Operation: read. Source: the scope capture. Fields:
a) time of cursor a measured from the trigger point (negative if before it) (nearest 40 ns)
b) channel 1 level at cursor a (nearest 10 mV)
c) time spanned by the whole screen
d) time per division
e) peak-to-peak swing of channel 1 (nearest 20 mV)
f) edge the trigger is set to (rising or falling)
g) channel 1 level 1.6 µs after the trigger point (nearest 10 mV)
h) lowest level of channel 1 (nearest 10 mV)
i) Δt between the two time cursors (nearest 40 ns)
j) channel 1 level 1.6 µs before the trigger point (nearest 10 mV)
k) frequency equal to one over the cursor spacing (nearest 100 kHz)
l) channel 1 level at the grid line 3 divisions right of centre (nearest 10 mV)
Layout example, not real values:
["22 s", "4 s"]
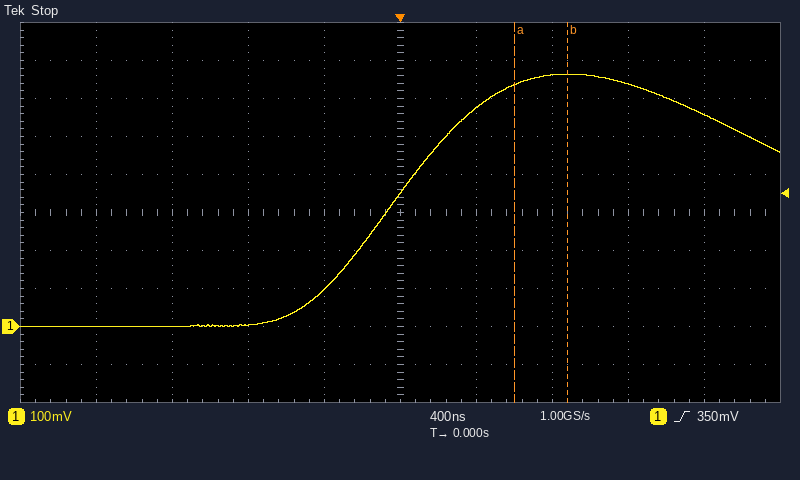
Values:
["+600 ns", "640 mV", "4 µs", "400 ns", "660 mV", "rising", "560 mV", "0 mV", "280 ns", "0 mV", "3.6 MHz", "640 mV"]
